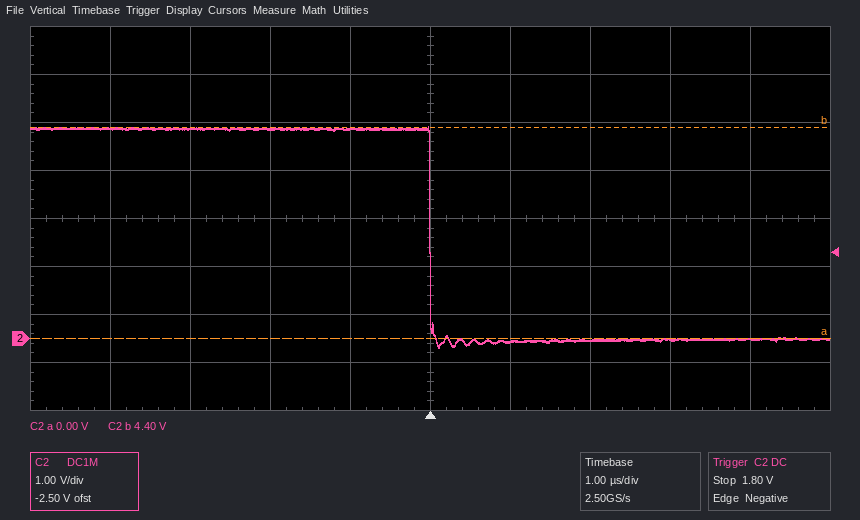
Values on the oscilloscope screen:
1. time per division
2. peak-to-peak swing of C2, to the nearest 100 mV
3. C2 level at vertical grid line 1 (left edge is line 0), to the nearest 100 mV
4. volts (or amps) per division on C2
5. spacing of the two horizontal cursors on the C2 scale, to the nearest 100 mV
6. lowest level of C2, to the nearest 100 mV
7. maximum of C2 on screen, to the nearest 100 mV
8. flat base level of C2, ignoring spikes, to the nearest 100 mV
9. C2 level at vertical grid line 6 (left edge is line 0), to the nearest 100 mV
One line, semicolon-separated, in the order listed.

1 µs; 4.6 V; 4.4 V; 1 V; 4.4 V; -200 mV; 4.4 V; 0.0 V; -100 mV
